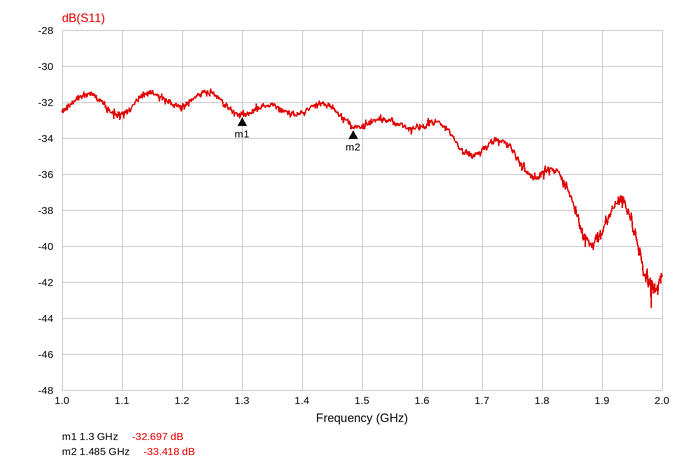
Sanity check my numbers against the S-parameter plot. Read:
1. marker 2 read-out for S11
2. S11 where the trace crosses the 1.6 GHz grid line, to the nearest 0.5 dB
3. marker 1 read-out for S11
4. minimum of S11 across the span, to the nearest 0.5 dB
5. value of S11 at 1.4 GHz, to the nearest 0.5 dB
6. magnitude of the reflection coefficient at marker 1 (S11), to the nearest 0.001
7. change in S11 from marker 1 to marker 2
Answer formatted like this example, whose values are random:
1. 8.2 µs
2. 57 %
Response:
1. -33.418 dB
2. -33.5 dB
3. -32.697 dB
4. -43.5 dB
5. -32.5 dB
6. 0.023
7. -0.721 dB
